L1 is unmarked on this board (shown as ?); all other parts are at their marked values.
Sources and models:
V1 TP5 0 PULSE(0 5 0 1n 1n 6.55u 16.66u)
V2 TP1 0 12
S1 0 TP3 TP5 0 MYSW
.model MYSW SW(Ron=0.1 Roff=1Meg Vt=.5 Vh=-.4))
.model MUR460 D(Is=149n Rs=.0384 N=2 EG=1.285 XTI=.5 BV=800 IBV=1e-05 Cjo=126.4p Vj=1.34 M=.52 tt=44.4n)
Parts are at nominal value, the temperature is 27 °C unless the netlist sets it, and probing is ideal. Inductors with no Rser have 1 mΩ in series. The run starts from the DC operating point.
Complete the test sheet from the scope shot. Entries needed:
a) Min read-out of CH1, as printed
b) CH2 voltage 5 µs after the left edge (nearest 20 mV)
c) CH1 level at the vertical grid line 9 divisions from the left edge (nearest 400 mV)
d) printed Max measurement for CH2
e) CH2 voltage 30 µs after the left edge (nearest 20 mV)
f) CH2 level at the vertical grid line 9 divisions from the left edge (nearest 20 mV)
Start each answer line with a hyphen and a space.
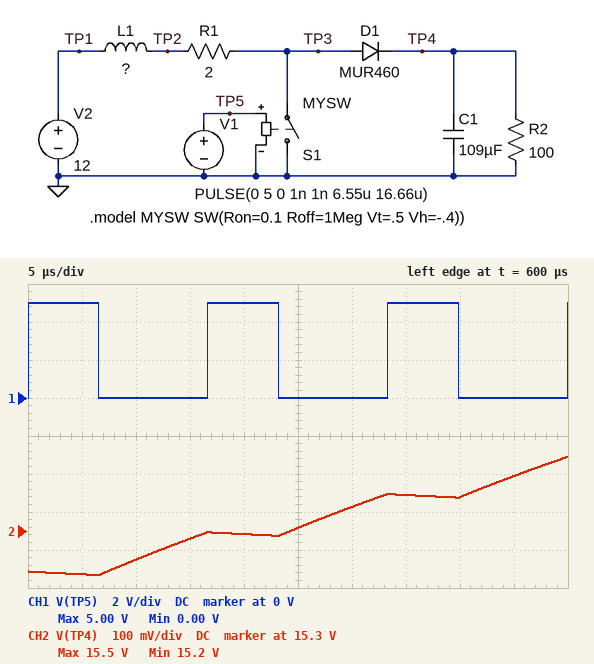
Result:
- 0.00 V
- 15.18 V
- 0 V
- 15.5 V
- 15.36 V
- 15.44 V
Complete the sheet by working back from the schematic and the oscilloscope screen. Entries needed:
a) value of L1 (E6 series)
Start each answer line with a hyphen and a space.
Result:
- 330 µH
